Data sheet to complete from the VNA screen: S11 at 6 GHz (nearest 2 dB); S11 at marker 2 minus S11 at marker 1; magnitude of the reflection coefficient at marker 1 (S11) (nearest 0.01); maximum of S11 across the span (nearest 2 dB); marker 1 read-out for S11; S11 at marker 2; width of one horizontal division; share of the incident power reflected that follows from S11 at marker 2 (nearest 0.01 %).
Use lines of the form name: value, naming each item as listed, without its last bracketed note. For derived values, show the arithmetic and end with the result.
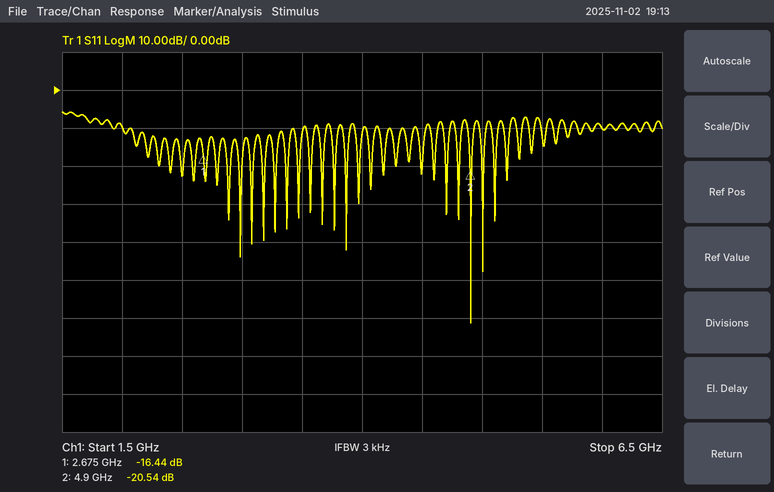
S11 at 6 GHz: -10 dB
S11 at marker 2 minus S11 at marker 1: -20.54 − (-16.44) = -4.10 dB
magnitude of the reflection coefficient at marker 1 (S11): 10^(-16.44/20) ≈ 0.15
maximum of S11 across the span: -6 dB
marker 1 read-out for S11: -16.44 dB
S11 at marker 2: -20.54 dB
width of one horizontal division: 500 MHz
share of the incident power reflected that follows from S11 at marker 2: 10^(-20.54/10) ≈ 0.88 %
